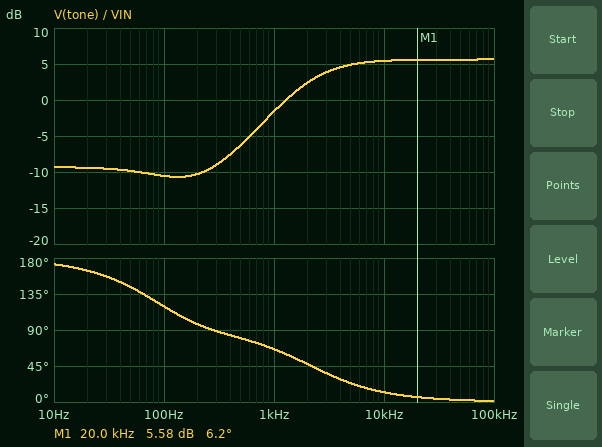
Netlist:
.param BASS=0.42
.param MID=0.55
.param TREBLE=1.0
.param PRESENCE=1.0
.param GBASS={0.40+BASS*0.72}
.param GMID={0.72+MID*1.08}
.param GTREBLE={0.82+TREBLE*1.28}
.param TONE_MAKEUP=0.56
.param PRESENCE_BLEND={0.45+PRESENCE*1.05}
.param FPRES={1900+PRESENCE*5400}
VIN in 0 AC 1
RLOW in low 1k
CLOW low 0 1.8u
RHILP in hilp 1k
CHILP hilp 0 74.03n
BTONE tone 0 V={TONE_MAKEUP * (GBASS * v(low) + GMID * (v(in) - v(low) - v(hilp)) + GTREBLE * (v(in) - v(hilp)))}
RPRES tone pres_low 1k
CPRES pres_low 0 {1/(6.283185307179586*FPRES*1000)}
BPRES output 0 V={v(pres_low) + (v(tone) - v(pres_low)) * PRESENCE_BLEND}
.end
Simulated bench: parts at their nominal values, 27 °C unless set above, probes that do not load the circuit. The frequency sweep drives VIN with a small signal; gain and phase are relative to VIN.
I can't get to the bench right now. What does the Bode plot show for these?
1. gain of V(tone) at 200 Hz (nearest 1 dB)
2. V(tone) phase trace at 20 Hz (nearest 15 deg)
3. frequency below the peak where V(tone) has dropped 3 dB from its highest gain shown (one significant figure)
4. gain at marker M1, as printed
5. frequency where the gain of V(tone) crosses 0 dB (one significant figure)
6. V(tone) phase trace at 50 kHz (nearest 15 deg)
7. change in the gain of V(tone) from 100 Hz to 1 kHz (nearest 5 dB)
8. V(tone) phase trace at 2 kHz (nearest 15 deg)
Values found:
-10 dB
165 deg
2 kHz
5.58 dB
1 kHz
0 deg
10 dB
45 deg
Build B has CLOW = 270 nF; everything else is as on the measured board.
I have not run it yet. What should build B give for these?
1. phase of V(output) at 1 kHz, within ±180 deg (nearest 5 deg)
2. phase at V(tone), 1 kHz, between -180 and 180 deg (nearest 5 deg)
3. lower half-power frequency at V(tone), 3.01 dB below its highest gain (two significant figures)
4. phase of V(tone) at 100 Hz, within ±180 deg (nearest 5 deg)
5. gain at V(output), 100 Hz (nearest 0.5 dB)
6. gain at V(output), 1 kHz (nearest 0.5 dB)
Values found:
80 deg
75 deg
2.0 kHz
155 deg
-9.0 dB
-0.5 dB
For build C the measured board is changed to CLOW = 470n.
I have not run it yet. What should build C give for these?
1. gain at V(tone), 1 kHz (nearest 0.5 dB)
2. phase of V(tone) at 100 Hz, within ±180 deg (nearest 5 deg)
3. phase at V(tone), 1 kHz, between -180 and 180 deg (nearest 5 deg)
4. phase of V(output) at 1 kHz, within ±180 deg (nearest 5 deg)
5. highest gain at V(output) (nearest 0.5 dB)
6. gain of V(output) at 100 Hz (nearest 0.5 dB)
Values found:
-1.0 dB
150 deg
70 deg
75 deg
9.0 dB
-9.0 dB
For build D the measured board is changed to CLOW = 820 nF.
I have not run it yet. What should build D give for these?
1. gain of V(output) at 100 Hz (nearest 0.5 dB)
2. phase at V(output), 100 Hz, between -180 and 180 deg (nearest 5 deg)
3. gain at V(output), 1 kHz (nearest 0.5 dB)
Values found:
-9.0 dB
140 deg
-1.0 dB
